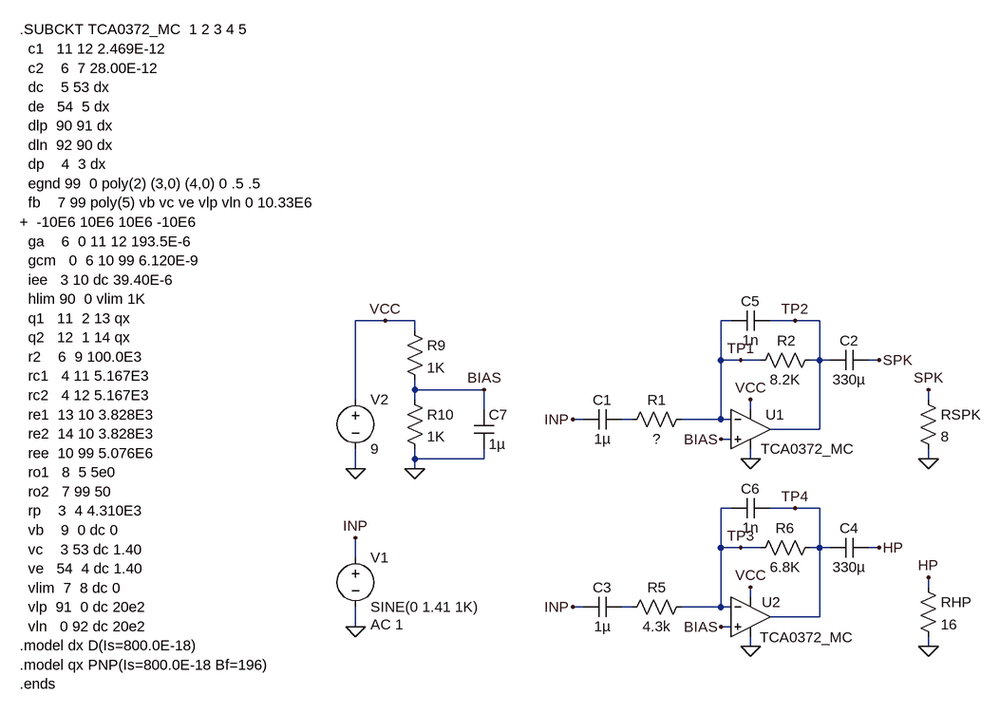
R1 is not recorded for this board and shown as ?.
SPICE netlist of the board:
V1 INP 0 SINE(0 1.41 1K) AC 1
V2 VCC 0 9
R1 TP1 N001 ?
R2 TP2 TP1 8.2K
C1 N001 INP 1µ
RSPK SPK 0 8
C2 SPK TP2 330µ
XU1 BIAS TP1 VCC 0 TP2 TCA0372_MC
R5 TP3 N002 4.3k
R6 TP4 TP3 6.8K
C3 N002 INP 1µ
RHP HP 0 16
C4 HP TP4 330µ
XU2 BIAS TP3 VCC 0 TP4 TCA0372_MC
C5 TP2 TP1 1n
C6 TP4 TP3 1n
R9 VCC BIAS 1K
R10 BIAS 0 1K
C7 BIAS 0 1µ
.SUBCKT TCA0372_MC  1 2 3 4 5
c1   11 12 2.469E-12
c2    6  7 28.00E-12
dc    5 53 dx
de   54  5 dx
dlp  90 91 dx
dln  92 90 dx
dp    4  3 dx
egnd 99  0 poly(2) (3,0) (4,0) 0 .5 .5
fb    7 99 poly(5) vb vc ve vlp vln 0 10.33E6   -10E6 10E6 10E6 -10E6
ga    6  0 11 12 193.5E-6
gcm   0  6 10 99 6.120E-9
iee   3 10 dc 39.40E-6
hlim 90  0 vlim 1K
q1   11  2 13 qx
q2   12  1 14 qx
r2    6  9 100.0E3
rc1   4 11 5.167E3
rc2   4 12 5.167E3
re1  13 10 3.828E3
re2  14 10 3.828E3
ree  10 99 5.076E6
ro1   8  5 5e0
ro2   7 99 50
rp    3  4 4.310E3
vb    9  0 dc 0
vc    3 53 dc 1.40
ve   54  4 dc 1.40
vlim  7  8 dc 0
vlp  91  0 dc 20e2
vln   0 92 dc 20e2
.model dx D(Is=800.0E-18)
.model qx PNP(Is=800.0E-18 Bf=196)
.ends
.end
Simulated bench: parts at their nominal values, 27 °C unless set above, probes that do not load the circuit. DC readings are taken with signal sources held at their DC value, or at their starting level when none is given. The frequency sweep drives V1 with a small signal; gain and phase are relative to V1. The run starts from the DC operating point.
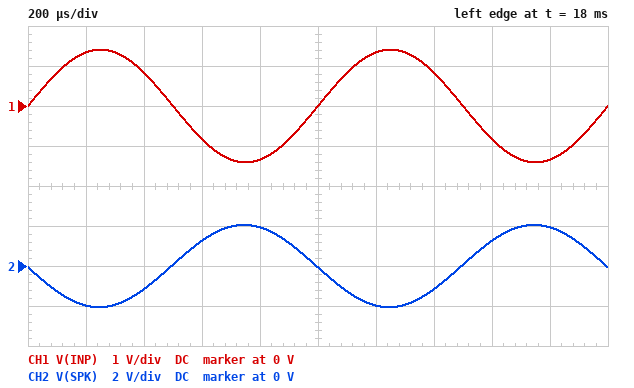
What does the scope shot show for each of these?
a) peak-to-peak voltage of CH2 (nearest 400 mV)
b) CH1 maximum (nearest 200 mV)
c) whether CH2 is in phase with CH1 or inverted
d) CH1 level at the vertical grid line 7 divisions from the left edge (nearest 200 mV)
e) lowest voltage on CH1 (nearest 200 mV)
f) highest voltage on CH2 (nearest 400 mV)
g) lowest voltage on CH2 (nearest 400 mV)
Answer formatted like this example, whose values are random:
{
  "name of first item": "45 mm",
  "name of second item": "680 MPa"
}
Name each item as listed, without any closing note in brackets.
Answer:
{
  "peak-to-peak voltage of CH2": "4.0 V",
  "CH1 maximum": "1.4 V",
  "whether CH2 is in phase with CH1 or inverted": "inverted",
  "CH1 level at the vertical grid line 7 divisions from the left edge": "800 mV",
  "lowest voltage on CH1": "-1.4 V",
  "highest voltage on CH2": "2.0 V",
  "lowest voltage on CH2": "-2.0 V"
}
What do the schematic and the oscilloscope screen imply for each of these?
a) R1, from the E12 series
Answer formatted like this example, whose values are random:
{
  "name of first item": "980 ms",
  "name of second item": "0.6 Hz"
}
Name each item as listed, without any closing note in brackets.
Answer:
{
  "R1, from the E12 series": "5.6 kΩ"
}
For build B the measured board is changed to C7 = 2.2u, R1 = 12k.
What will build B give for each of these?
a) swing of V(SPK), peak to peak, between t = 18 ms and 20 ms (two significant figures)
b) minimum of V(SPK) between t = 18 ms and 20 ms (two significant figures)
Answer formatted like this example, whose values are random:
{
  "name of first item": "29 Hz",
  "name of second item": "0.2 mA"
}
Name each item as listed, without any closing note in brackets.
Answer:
{
  "swing of V(SPK), peak to peak, between t = 18 ms and 20 ms": "1.9 V",
  "minimum of V(SPK) between t = 18 ms and 20 ms": "-960 mV"
}
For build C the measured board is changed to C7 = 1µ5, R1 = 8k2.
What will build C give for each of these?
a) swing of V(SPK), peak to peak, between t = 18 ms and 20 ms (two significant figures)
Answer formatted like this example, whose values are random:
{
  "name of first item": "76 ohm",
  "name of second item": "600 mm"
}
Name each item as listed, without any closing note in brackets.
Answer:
{
  "swing of V(SPK), peak to peak, between t = 18 ms and 20 ms": "2.8 V"
}
